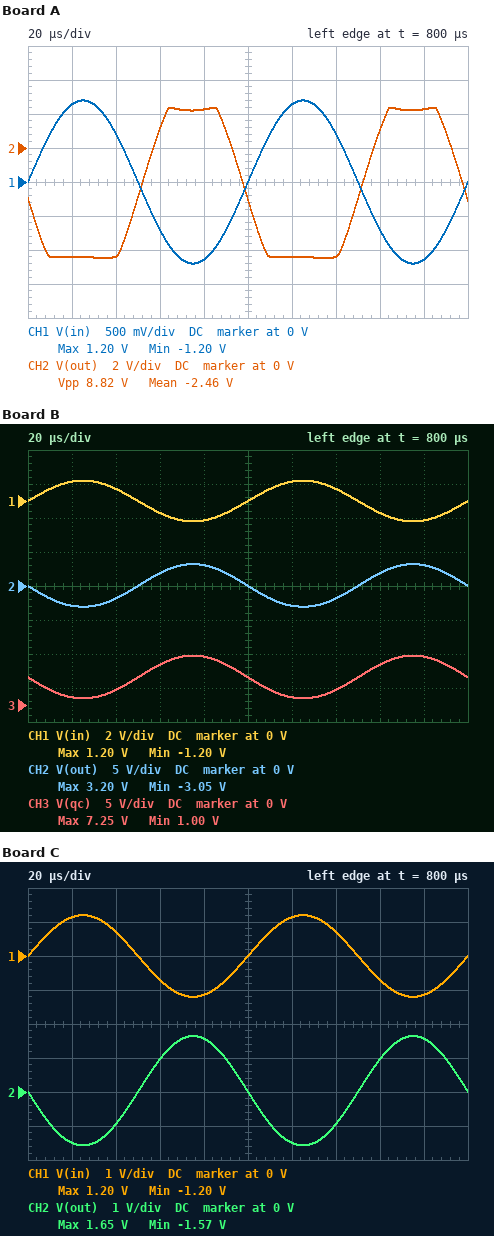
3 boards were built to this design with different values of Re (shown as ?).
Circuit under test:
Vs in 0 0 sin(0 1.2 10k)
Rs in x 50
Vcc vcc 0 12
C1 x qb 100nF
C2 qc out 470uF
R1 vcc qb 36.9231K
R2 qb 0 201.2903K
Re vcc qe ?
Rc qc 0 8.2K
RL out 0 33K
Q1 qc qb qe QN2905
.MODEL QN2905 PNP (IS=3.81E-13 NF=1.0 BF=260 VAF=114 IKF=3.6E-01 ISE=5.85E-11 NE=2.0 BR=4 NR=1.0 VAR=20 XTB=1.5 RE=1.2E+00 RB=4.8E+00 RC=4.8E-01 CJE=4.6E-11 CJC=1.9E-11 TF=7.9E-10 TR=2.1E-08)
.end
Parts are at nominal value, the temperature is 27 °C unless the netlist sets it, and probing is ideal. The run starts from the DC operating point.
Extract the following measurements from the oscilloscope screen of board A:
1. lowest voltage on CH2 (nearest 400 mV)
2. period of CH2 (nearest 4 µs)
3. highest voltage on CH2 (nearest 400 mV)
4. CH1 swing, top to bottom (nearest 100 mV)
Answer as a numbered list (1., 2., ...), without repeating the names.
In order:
1. -6.4 V
2. 100 µs
3. 2.4 V
4. 2.4 V
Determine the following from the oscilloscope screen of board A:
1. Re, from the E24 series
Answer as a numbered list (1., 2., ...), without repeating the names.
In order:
1. 1.1 kΩ
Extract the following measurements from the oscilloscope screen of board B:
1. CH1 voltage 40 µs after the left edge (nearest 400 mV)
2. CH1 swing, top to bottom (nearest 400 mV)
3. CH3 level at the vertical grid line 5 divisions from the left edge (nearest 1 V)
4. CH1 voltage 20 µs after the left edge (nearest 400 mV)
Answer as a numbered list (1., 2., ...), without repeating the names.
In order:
1. 800 mV
2. 2.4 V
3. 4 V
4. 1.2 V
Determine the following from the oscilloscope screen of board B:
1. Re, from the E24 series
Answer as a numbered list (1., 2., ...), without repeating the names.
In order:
1. 2.4 kΩ
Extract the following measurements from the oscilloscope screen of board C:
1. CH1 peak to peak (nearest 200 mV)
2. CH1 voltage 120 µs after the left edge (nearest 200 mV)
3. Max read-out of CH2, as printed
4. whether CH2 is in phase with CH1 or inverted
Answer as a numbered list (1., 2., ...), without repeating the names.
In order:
1. 2.4 V
2. 1.2 V
3. 1.65 V
4. inverted
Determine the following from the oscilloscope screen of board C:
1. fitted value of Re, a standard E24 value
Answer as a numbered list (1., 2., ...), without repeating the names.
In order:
1. 4.7 kΩ
